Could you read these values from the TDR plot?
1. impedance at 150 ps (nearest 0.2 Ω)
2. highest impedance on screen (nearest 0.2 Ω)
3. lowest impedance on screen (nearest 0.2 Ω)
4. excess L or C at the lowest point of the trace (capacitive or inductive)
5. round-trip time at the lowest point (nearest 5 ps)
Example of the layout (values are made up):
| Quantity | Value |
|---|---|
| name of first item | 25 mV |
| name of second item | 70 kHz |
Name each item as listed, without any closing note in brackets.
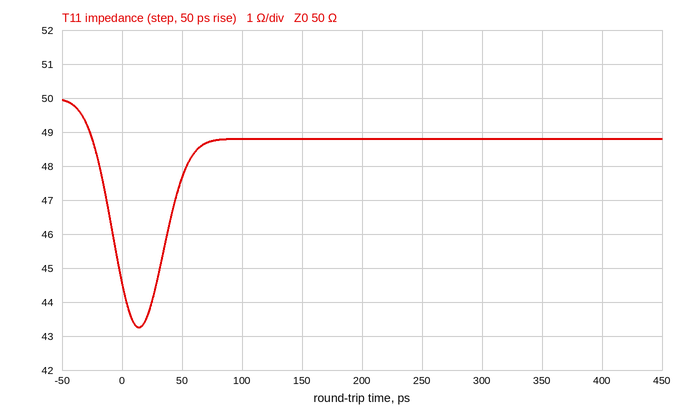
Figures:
| Quantity | Value |
|---|---|
| impedance at 150 ps | 48.8 Ω |
| highest impedance on screen | 50.0 Ω |
| lowest impedance on screen | 43.2 Ω |
| excess L or C at the lowest point of the trace | capacitive |
| round-trip time at the lowest point | 15 ps |
